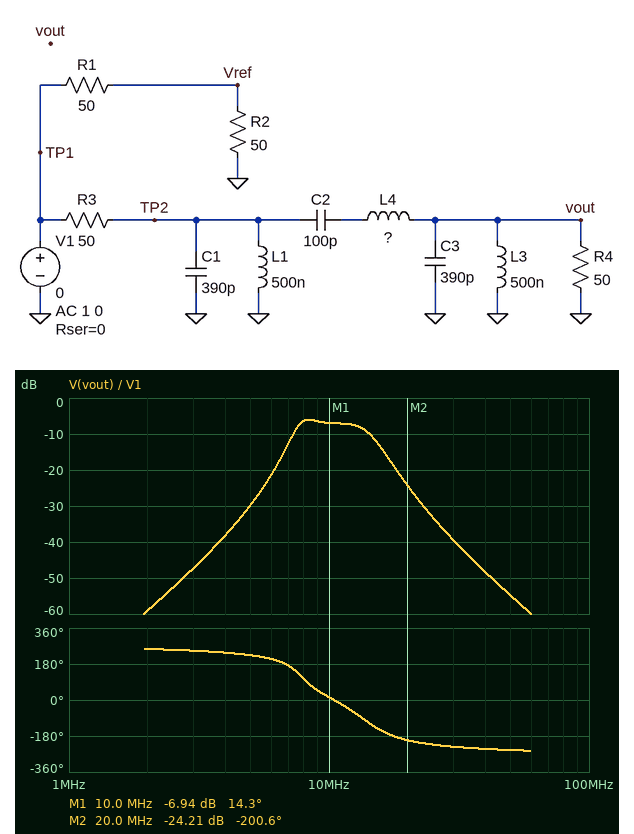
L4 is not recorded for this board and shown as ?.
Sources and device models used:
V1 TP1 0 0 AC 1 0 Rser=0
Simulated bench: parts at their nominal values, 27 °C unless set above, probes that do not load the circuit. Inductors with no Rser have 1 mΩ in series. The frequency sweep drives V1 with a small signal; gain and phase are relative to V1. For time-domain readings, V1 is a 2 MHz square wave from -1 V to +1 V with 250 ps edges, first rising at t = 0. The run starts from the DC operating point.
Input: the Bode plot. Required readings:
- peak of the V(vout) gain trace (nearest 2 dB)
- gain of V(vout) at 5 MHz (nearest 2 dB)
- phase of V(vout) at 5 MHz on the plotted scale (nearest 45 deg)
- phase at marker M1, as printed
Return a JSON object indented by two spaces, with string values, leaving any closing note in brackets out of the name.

{
  "peak of the V(vout) gain trace": "-6 dB",
  "gain of V(vout) at 5 MHz": "-30 dB",
  "phase of V(vout) at 5 MHz on the plotted scale": "225 deg",
  "phase at marker M1, as printed": "14.3 deg"
}
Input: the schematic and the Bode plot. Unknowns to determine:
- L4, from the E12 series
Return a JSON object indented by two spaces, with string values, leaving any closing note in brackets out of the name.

{
  "L4, from the E12 series": "2.7 µH"
}
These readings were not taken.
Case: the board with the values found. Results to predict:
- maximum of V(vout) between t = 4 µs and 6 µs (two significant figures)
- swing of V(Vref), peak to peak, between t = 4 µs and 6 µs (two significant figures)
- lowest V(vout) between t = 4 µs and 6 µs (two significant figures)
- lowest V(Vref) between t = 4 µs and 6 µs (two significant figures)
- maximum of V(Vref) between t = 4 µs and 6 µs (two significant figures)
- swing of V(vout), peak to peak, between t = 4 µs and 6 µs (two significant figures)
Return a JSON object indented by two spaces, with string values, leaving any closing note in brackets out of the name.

{
  "maximum of V(vout) between t = 4 µs and 6 µs": "190 mV",
  "swing of V(Vref), peak to peak, between t = 4 µs and 6 µs": "1.0 V",
  "lowest V(vout) between t = 4 µs and 6 µs": "-190 mV",
  "lowest V(Vref) between t = 4 µs and 6 µs": "-500 mV",
  "maximum of V(Vref) between t = 4 µs and 6 µs": "500 mV",
  "swing of V(vout), peak to peak, between t = 4 µs and 6 µs": "390 mV"
}
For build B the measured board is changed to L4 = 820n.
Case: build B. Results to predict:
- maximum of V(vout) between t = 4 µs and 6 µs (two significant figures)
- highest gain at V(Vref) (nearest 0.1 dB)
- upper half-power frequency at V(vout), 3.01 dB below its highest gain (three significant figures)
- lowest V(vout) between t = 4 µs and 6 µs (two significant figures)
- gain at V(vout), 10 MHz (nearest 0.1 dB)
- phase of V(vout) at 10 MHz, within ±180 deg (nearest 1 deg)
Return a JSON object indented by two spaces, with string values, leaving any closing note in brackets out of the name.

{
  "maximum of V(vout) between t = 4 µs and 6 µs": "290 mV",
  "highest gain at V(Vref)": "-6.0 dB",
  "upper half-power frequency at V(vout), 3.01 dB below its highest gain": "23.6 MHz",
  "lowest V(vout) between t = 4 µs and 6 µs": "-290 mV",
  "gain at V(vout), 10 MHz": "-8.4 dB",
  "phase of V(vout) at 10 MHz, within ±180 deg": "81 deg"
}
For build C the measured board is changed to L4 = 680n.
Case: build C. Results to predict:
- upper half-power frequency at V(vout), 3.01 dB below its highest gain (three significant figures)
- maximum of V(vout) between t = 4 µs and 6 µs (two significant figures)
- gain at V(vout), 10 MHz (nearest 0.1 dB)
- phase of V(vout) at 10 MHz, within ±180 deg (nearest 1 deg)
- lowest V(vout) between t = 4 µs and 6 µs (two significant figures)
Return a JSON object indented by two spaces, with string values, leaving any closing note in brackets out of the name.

{
  "upper half-power frequency at V(vout), 3.01 dB below its highest gain": "25.7 MHz",
  "maximum of V(vout) between t = 4 µs and 6 µs": "260 mV",
  "gain at V(vout), 10 MHz": "-8.8 dB",
  "phase of V(vout) at 10 MHz, within ±180 deg": "84 deg",
  "lowest V(vout) between t = 4 µs and 6 µs": "-260 mV"
}
